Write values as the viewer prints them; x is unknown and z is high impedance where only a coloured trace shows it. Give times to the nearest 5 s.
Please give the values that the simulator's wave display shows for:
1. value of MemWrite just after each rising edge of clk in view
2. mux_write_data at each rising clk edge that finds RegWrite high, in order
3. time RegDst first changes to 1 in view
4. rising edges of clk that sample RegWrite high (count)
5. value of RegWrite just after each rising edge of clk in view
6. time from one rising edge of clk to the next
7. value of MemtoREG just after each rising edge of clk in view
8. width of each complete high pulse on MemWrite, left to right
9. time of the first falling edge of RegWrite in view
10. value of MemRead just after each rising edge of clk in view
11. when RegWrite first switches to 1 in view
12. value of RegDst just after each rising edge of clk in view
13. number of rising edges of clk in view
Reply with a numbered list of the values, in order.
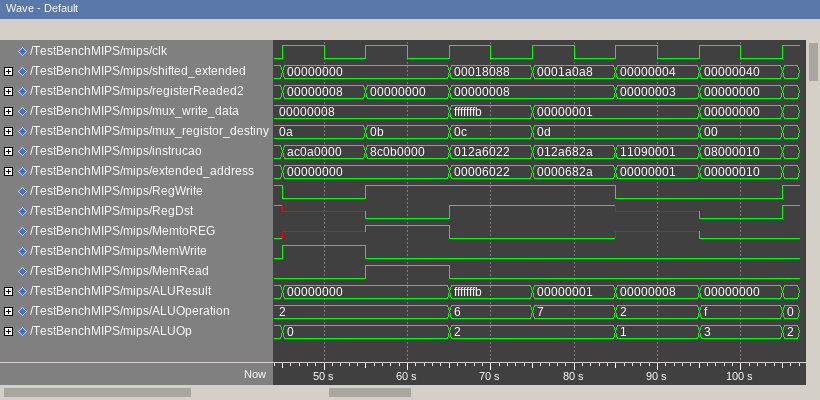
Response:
1. 1 0 0 0 0 0 0
2. 00000008, 00000008, fffffffb, 00000001
3. 65 s
4. 4
5. 0 1 1 1 0 0 1
6. 10 s
7. x 1 0 0 x 0 0
8. 10 s
9. 45 s
10. 0 1 0 0 0 0 0
11. 55 s
12. x 0 1 1 x 0 1
13. 7
